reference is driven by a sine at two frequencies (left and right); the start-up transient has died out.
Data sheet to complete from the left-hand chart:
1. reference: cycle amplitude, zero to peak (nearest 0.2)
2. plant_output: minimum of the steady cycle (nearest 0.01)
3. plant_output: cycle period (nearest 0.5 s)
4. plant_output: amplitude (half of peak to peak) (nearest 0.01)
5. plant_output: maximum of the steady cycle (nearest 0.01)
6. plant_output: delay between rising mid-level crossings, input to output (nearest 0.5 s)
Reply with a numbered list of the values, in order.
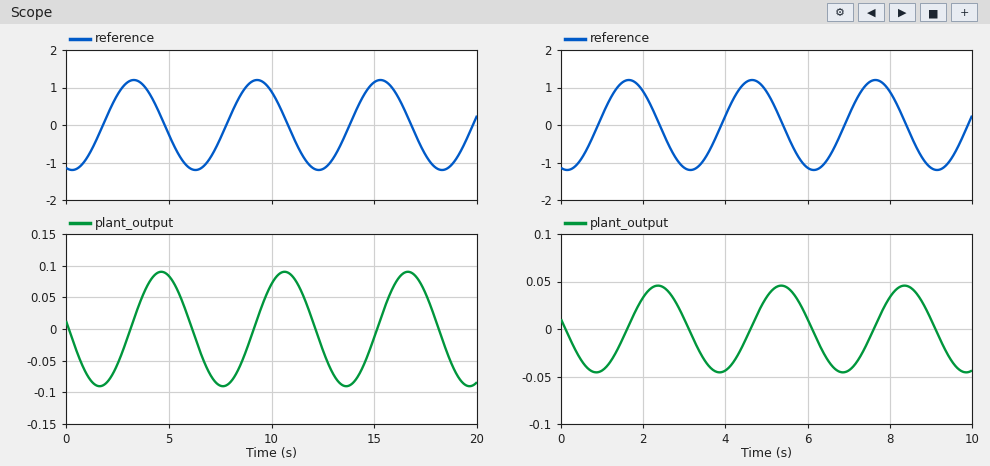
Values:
1. 1.2
2. -0.09
3. 6.0 s
4. 0.09
5. 0.09
6. 1.5 s
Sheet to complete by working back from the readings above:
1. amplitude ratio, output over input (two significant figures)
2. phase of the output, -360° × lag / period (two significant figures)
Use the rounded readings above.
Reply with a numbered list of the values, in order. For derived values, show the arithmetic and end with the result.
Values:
1. 0.09 / 1.2 = 0.075
2. -360 × 1.5 / 6 = -90°
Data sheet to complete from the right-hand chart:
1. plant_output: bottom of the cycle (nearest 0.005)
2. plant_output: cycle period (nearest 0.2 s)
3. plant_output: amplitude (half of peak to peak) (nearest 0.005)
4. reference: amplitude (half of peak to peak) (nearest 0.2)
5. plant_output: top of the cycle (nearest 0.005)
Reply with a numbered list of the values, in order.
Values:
1. -0.045
2. 3.0 s
3. 0.045
4. 1.2
5. 0.045
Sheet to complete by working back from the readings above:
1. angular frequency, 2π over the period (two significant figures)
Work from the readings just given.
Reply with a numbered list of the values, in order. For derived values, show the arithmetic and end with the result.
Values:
1. 2π / 3 = 2.1 rad/s
